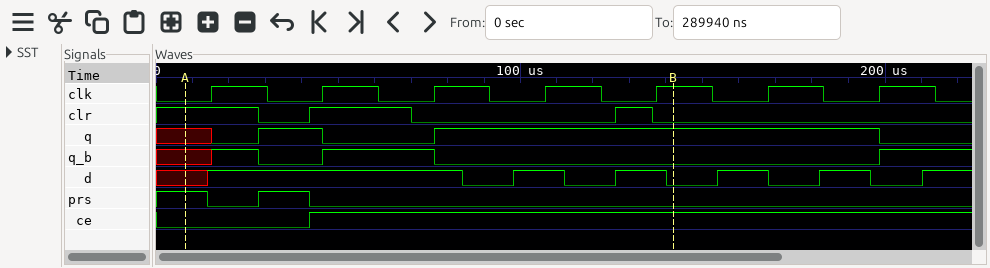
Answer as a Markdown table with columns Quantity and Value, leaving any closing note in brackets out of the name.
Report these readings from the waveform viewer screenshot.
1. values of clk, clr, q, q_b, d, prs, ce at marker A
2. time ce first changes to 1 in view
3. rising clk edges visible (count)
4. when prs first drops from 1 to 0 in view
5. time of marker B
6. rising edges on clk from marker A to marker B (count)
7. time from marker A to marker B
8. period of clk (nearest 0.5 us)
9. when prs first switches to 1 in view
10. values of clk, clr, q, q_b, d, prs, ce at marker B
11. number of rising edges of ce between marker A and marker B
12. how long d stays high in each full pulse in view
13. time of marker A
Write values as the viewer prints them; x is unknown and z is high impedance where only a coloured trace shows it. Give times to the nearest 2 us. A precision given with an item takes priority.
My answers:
| Quantity | Value |
|---|---|
| values of clk, clr, q, q_b, d, prs, ce at marker A | clk=0, clr=1, q=x, q_b=x, d=x, prs=1, ce=0 |
| time ce first changes to 1 in view | 42 us |
| rising clk edges visible | 7 |
| when prs first drops from 1 to 0 in view | 14 us |
| time of marker B | 142 us |
| rising edges on clk from marker A to marker B | 5 |
| time from marker A to marker B | 134 us |
| period of clk | 30.5 us |
| when prs first switches to 1 in view | 28 us |
| values of clk, clr, q, q_b, d, prs, ce at marker B | clk=1, clr=0, q=1, q_b=0, d=0, prs=0, ce=1 |
| number of rising edges of ce between marker A and marker B | 1 |
| how long d stays high in each full pulse in view | 14 us, 14 us, 14 us, 14 us |
| time of marker A | 8 us |
